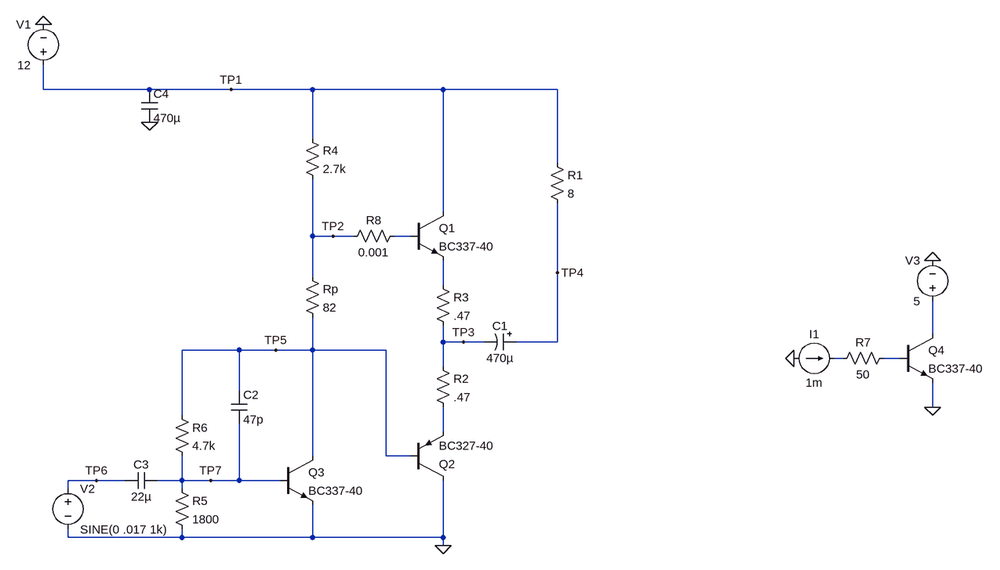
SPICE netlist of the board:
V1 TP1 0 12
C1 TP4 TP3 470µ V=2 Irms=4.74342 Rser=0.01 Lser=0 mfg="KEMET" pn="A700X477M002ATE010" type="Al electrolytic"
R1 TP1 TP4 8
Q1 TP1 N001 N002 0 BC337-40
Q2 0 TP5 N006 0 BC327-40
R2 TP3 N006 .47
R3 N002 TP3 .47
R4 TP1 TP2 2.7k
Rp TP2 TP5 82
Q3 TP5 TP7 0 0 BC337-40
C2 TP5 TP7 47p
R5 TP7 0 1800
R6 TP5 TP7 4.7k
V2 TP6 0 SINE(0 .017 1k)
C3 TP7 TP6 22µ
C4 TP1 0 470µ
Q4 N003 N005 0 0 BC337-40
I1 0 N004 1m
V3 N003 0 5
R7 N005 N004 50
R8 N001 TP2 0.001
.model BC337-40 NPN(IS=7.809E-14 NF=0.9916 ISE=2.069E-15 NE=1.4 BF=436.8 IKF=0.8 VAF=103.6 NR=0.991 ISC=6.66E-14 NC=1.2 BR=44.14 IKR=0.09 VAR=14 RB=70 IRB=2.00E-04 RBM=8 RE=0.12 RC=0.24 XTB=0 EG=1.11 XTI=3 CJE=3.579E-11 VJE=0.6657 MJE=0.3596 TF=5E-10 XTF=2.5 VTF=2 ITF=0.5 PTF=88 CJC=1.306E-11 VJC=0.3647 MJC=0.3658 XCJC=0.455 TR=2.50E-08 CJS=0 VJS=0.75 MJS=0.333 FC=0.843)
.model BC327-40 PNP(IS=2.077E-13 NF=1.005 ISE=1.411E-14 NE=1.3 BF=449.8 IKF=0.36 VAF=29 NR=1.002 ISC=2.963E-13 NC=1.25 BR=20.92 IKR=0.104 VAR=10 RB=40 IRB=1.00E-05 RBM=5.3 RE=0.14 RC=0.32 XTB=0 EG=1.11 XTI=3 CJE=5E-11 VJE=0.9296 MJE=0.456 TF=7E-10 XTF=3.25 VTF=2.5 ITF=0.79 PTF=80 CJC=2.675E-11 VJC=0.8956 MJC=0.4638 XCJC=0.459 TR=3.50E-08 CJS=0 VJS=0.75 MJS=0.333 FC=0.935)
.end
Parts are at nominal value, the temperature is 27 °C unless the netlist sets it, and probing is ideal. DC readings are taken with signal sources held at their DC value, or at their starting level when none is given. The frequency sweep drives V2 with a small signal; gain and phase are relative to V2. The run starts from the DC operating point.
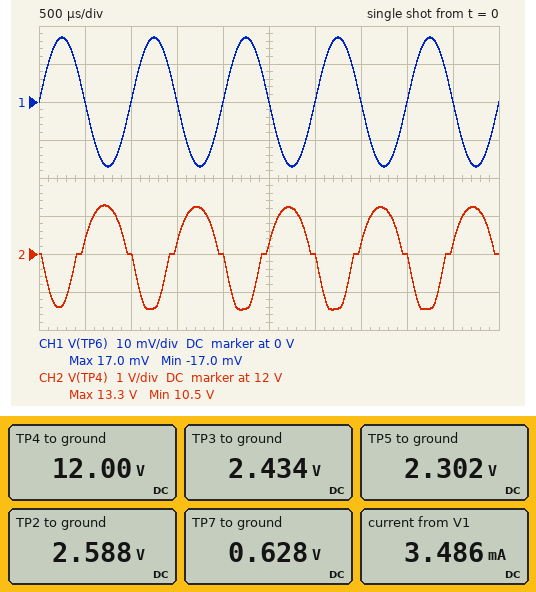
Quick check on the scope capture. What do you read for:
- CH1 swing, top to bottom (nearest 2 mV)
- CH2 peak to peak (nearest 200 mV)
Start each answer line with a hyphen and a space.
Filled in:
- 34 mV
- 2.8 V
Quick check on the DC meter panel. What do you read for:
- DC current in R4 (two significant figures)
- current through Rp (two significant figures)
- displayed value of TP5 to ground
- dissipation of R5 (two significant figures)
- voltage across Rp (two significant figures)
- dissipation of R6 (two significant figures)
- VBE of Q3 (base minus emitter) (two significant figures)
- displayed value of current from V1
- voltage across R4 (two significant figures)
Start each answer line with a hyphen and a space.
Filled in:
- 3.5 mA
- 3.5 mA
- 2.302 V
- 220 µW
- 290 mV
- 600 µW
- 630 mV
- 3.486 mA
- 9.4 V
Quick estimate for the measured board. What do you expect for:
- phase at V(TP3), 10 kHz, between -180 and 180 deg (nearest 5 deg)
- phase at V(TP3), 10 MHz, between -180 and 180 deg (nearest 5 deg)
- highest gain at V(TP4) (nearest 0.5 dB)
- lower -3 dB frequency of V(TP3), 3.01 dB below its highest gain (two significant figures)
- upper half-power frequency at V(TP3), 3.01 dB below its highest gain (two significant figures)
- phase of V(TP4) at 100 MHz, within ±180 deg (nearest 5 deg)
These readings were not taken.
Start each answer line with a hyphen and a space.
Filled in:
- -90 deg
- 145 deg
- -7.0 dB
- 480 kHz
- 21 MHz
- 40 deg
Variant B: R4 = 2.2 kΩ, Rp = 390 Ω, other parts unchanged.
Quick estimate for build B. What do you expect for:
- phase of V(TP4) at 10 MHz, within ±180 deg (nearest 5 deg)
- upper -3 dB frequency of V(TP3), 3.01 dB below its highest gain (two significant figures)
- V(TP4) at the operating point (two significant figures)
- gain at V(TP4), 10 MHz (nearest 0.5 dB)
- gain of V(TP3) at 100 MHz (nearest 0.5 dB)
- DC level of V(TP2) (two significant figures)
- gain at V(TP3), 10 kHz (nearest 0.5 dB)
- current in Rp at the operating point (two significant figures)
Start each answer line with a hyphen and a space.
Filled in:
- 60 deg
- 820 kHz
- 12 V
- 18.5 dB
- -8.0 dB
- 3.7 V
- 41.0 dB
- 3.7 mA
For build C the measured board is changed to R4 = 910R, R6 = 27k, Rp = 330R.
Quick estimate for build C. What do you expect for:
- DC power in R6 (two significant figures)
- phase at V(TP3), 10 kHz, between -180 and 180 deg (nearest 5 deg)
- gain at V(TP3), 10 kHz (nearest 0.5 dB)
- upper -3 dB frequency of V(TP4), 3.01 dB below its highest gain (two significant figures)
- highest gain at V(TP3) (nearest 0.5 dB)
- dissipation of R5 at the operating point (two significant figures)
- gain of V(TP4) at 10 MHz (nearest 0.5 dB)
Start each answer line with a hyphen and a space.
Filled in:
- 3.1 mW
- -100 deg
- -50.5 dB
- 25 MHz
- -12.0 dB
- 200 µW
- -13.0 dB
